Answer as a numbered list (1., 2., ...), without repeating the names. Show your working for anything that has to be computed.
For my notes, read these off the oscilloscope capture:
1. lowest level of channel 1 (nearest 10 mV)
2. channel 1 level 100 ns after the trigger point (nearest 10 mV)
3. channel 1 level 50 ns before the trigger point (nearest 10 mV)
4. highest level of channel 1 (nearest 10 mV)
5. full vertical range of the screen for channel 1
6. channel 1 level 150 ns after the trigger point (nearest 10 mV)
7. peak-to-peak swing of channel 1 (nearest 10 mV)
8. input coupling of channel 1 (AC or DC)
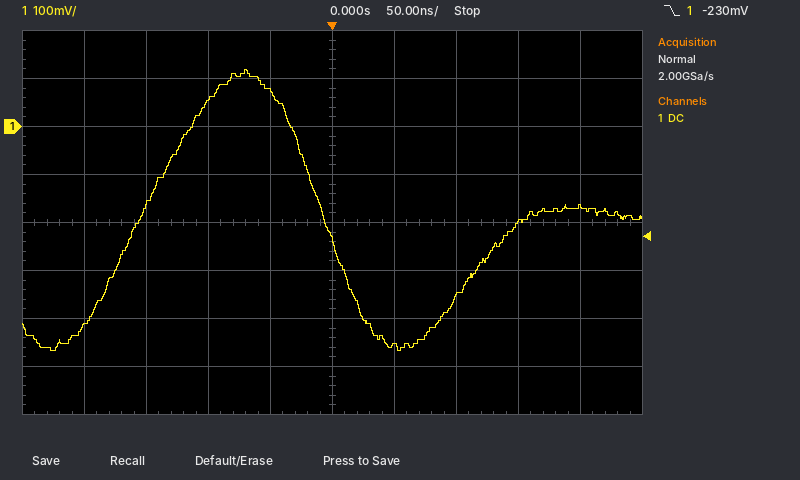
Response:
1. -470 mV
2. -360 mV
3. 70 mV
4. 120 mV
5. 800 mV
6. -200 mV
7. 120 mV − (-470 mV) = 590 mV
8. DC
